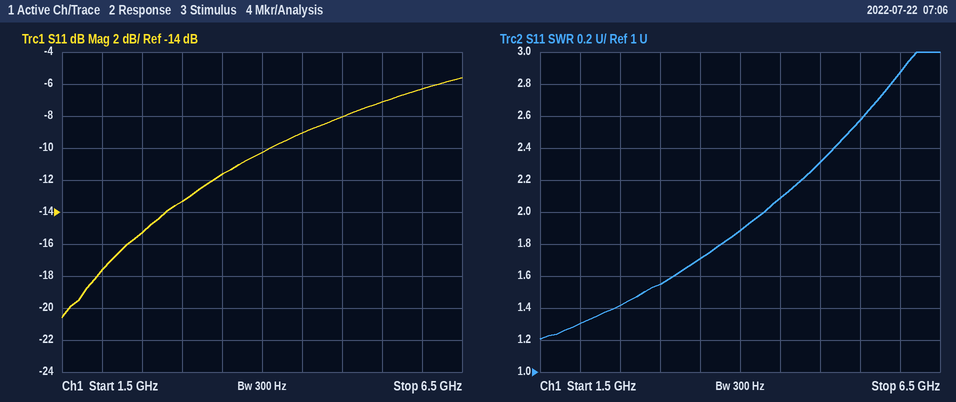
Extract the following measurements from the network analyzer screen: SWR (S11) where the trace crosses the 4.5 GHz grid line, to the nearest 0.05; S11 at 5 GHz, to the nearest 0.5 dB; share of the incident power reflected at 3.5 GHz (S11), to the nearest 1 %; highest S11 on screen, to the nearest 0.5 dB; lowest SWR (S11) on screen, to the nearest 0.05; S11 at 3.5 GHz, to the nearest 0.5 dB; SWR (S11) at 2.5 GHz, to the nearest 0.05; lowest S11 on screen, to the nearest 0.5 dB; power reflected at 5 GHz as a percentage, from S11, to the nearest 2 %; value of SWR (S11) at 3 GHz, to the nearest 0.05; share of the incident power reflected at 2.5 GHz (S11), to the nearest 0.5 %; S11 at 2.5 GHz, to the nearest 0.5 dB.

2.10
-8.0 dB
7 %
-5.5 dB
1.20
-11.5 dB
1.40
-20.5 dB
16 %
1.55
3.0 %
-15.5 dB
